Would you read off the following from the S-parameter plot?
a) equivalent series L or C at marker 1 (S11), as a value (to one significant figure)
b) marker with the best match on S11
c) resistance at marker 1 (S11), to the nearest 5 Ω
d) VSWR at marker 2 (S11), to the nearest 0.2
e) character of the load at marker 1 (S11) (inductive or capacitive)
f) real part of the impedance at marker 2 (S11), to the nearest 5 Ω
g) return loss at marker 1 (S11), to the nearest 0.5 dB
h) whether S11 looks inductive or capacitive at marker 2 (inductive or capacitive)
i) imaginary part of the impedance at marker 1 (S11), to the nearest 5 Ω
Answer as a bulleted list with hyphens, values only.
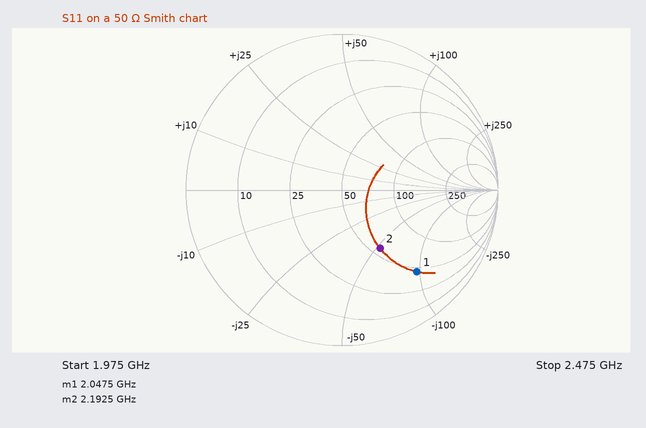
- 800 fF
- marker 2
- 45 Ω
- 2.6
- capacitive
- 55 Ω
- 3.0 dB
- capacitive
- -95 Ω
